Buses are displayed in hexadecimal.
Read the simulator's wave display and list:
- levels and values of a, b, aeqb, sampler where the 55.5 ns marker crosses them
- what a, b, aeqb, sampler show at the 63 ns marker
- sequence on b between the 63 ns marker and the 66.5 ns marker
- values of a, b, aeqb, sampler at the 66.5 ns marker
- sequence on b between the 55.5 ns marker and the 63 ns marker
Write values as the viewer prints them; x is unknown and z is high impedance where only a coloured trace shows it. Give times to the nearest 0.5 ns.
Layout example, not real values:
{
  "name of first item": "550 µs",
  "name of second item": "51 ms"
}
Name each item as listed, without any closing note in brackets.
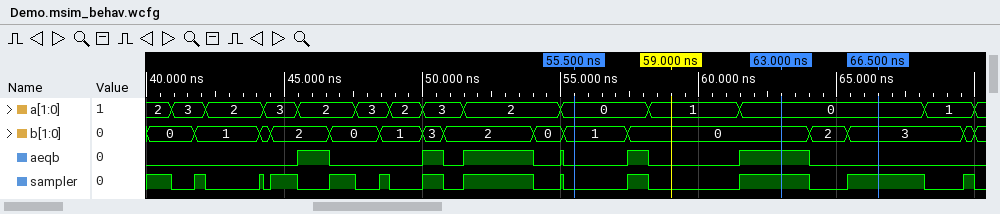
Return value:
{
  "levels and values of a, b, aeqb, sampler where the 55.5 ns marker crosses them": "a=0, b=1, aeqb=0, sampler=0",
  "what a, b, aeqb, sampler show at the 63 ns marker": "a=0, b=0, aeqb=1, sampler=1",
  "sequence on b between the 63 ns marker and the 66.5 ns marker": "0, 2, 3",
  "values of a, b, aeqb, sampler at the 66.5 ns marker": "a=0, b=3, aeqb=0, sampler=1",
  "sequence on b between the 55.5 ns marker and the 63 ns marker": "1, 0"
}
